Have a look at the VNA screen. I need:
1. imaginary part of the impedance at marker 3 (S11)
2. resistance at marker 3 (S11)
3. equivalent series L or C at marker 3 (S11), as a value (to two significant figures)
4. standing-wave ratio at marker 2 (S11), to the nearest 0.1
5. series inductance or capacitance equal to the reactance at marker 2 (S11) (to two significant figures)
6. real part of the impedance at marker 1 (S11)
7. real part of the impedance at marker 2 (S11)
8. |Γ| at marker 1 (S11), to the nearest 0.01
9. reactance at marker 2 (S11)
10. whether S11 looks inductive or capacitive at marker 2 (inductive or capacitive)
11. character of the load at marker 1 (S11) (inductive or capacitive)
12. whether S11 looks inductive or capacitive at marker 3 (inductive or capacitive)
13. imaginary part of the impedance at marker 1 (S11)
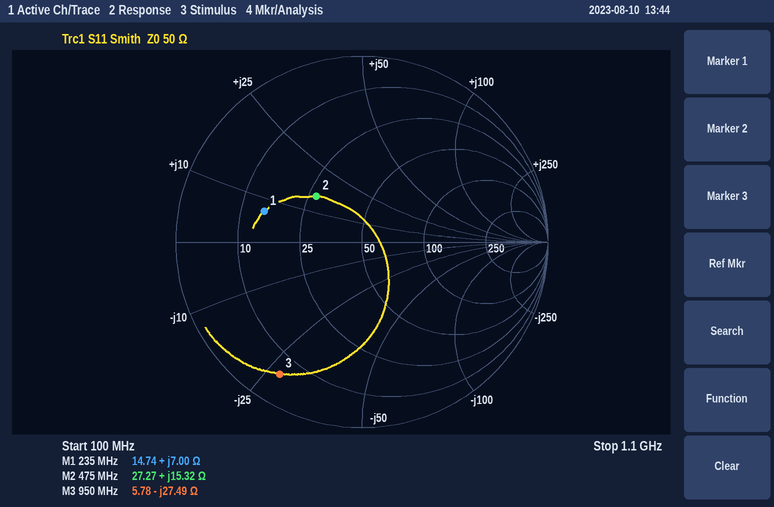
-27.49 Ω
5.78 Ω
6.1 pF
2.1
5.1 nH
14.74 Ω
27.27 Ω
0.55
+15.32 Ω
inductive
inductive
capacitive
+7.00 Ω
